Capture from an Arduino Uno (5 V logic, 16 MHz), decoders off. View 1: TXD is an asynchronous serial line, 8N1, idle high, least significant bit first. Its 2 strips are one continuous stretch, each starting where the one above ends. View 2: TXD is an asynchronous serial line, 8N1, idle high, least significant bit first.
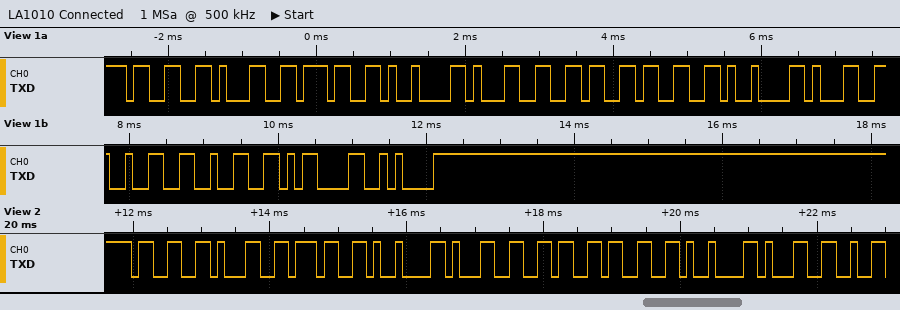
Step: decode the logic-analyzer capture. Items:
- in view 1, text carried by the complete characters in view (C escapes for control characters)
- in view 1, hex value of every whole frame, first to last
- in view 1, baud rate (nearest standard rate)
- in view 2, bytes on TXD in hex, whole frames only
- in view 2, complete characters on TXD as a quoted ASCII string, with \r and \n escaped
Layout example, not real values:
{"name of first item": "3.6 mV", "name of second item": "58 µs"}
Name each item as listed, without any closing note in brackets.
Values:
{"in view 1, text carried by the complete characters in view": "\"317\\t163\\t122\\r\\n\"", "in view 1, hex value of every whole frame, first to last": "0x33 0x31 0x37 0x09 0x31 0x36 0x33 0x09 0x31 0x32 0x32 0x0D 0x0A", "in view 1, baud rate": "9600 baud", "in view 2, bytes on TXD in hex, whole frames only": "0x33 0x31 0x37 0x09 0x31 0x36 0x33 0x09 0x31", "in view 2, complete characters on TXD as a quoted ASCII string, with \\r and \\n escaped": "\"317\\t163\\t1\""}
